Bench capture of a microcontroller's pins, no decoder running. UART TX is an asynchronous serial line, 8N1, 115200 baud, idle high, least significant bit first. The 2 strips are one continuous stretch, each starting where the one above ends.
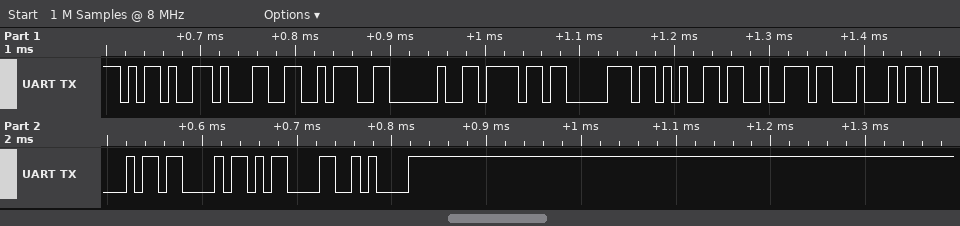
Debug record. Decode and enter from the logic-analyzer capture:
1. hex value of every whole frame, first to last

0x2D 0x31 0x3A 0x20 0x6F 0x70 0x65 0x72 0x44 0x41 0x43 0x0D 0x0A
